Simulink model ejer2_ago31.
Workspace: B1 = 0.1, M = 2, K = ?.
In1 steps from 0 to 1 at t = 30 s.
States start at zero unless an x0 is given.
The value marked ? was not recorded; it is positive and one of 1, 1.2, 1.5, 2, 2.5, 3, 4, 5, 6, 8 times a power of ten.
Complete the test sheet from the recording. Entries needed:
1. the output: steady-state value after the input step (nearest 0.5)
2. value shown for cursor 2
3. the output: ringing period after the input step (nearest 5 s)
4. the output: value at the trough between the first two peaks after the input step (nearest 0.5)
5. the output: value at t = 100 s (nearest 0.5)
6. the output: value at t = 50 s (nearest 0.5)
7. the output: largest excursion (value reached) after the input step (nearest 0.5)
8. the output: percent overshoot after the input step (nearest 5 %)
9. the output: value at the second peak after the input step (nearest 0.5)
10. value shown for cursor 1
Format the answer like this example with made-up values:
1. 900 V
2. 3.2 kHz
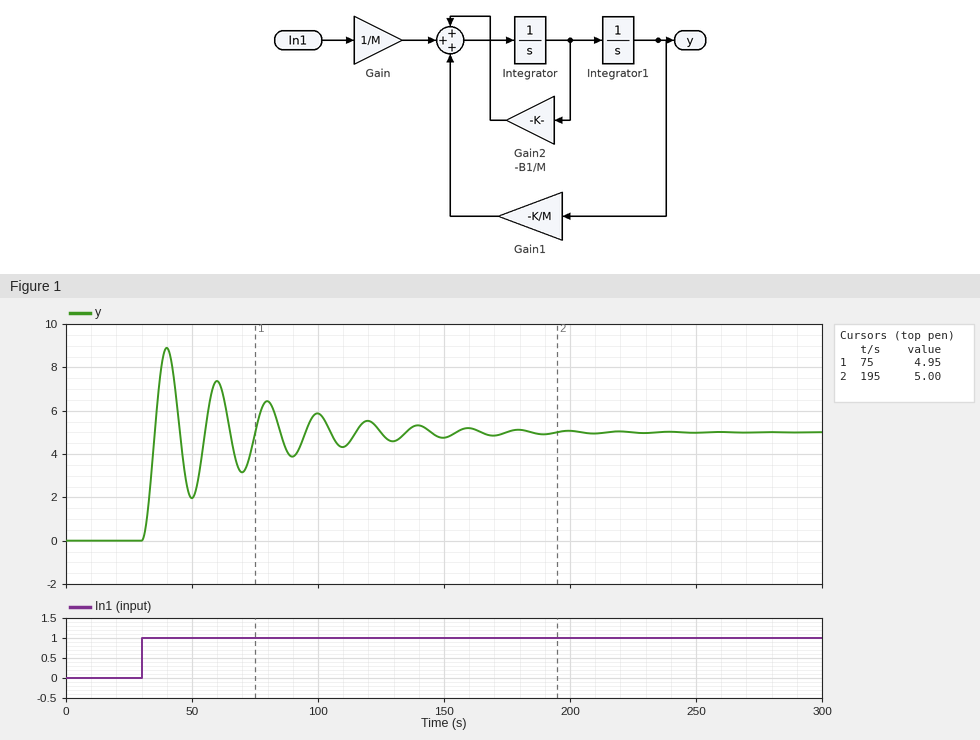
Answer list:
1. 5.0
2. 5.00
3. 20 s
4. 2.0
5. 6.0
6. 2.0
7. 9.0
8. 80 %
9. 7.5
10. 4.95
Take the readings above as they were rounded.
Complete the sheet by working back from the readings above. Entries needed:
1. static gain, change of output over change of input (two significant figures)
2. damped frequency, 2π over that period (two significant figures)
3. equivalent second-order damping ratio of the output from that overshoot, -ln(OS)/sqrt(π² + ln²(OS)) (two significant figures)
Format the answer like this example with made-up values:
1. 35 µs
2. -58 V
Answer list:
1. 5.0
2. 0.31 rad/s
3. 0.071
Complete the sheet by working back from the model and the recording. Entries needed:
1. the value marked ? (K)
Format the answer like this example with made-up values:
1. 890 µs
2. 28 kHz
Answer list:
1. 0.2
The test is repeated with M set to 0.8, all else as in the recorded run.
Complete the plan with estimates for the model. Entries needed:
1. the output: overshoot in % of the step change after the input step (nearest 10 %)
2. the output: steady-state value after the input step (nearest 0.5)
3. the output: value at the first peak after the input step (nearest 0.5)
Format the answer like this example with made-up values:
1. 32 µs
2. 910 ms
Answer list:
1. 70 %
2. 5.0
3. 8.5
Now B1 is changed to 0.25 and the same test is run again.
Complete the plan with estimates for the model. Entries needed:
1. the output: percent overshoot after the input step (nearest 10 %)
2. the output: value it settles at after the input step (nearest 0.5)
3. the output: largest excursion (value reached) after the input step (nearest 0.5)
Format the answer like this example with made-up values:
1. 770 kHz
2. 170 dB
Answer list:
1. 50 %
2. 5.0
3. 7.5
